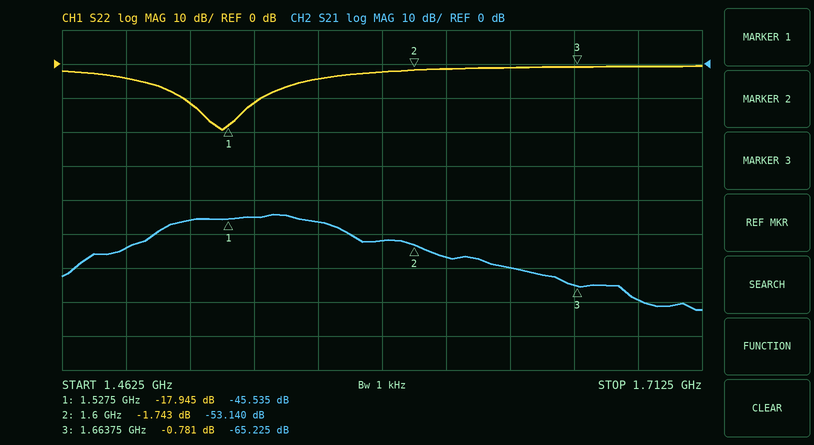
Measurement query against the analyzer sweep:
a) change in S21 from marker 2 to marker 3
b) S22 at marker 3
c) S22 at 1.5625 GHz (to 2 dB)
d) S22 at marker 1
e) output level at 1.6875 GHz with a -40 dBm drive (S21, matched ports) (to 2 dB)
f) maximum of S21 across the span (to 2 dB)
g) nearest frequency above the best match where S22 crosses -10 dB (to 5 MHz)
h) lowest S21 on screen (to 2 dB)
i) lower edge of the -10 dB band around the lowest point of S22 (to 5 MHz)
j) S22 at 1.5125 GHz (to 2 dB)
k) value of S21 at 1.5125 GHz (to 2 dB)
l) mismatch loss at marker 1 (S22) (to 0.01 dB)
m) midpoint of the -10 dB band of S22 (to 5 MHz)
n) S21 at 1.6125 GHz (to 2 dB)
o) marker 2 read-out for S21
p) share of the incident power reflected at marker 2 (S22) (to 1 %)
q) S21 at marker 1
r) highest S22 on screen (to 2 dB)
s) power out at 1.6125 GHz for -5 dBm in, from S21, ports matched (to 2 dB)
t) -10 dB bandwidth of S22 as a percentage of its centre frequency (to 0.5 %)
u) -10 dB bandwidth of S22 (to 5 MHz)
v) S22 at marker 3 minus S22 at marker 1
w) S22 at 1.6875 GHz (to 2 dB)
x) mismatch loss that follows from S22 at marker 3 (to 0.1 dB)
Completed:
-12.085 dB
-0.781 dB
-4 dB
-17.945 dB
-110 dBm
-44 dB
1.540 GHz
-72 dB
1.510 GHz
-12 dB
-46 dB
0.07 dB
1.525 GHz
-56 dB
-53.140 dB
67 %
-45.535 dB
0 dB
-62 dBm
2.0 %
30 MHz
17.164 dB
0 dB
7.8 dB
